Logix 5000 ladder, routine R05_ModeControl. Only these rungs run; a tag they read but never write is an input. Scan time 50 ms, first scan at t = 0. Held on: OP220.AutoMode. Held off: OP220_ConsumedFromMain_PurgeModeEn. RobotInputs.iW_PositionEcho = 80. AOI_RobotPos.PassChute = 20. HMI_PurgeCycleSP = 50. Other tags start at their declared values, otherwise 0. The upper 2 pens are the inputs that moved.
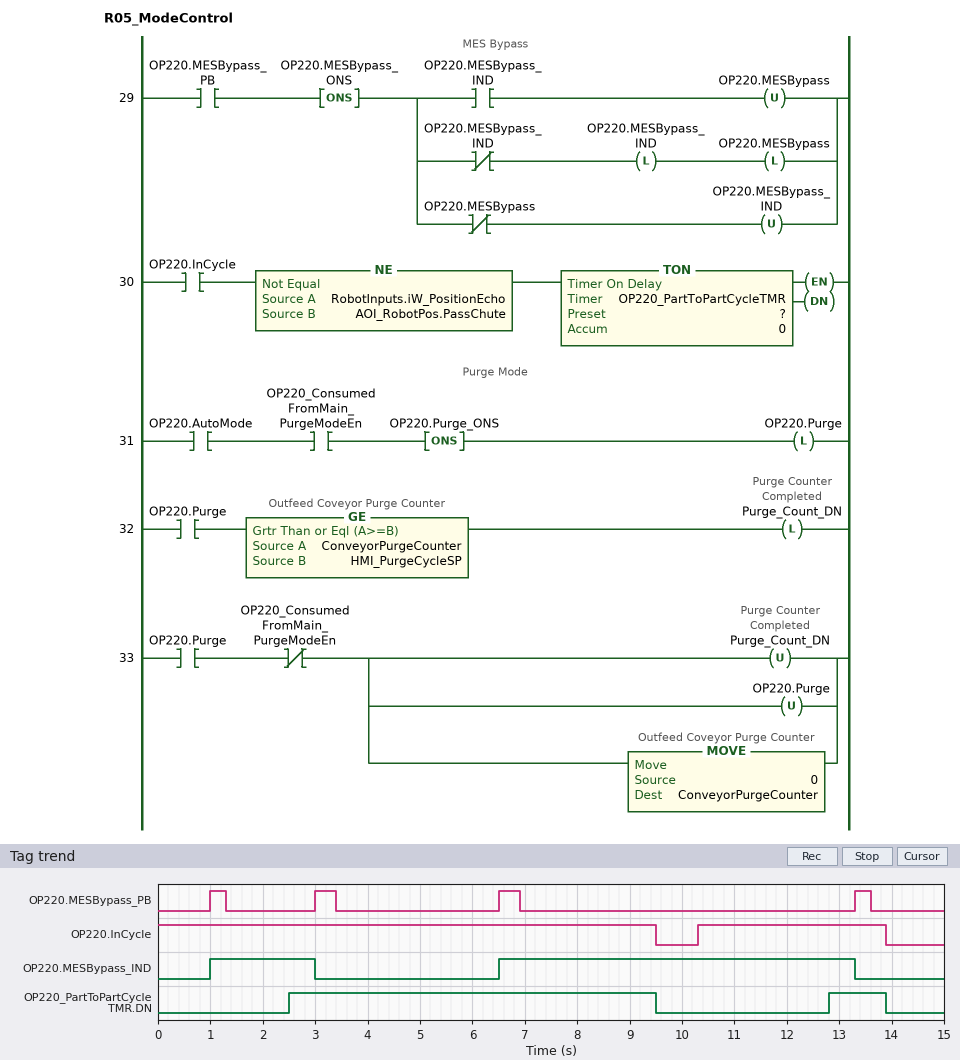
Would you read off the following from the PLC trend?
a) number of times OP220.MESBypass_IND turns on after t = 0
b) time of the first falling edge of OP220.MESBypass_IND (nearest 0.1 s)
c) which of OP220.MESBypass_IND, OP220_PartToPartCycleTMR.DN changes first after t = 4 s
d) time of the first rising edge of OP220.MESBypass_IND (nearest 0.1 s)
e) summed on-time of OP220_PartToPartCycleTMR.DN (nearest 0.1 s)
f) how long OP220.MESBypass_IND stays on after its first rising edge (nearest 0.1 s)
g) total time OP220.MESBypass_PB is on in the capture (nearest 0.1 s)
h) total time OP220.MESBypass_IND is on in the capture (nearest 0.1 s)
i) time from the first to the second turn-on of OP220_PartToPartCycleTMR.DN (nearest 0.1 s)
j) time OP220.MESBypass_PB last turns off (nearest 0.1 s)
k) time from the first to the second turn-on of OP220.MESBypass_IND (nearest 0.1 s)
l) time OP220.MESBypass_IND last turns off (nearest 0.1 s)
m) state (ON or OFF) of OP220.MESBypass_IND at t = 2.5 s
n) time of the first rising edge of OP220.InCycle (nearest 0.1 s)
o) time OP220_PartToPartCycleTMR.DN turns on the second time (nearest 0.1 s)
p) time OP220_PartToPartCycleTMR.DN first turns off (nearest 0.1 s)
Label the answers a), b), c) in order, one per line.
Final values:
a) 2
b) 3.0 s
c) OP220.MESBypass_IND
d) 1.0 s
e) 8.1 s
f) 2.0 s
g) 1.4 s
h) 8.8 s
i) 10.3 s
j) 13.6 s
k) 5.5 s
l) 13.3 s
m) ON
n) 10.3 s
o) 12.8 s
p) 9.5 s
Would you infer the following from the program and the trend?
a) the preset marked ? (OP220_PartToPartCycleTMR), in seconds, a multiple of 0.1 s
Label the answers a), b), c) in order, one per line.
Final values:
a) 2.5 s
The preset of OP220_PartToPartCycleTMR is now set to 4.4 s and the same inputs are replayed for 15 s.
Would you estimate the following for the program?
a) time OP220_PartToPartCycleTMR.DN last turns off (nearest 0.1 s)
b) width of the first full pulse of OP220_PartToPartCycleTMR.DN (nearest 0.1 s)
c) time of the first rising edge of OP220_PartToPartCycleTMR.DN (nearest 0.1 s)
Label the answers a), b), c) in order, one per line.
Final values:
a) 9.5 s
b) 5.1 s
c) 4.4 s
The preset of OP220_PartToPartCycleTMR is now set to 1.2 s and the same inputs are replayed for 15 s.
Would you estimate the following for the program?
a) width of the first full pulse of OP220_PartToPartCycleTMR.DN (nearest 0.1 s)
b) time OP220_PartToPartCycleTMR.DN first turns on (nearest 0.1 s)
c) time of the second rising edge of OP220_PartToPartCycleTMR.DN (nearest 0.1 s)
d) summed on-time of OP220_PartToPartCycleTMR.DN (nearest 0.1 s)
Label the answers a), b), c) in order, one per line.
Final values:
a) 8.3 s
b) 1.2 s
c) 11.5 s
d) 10.7 s
